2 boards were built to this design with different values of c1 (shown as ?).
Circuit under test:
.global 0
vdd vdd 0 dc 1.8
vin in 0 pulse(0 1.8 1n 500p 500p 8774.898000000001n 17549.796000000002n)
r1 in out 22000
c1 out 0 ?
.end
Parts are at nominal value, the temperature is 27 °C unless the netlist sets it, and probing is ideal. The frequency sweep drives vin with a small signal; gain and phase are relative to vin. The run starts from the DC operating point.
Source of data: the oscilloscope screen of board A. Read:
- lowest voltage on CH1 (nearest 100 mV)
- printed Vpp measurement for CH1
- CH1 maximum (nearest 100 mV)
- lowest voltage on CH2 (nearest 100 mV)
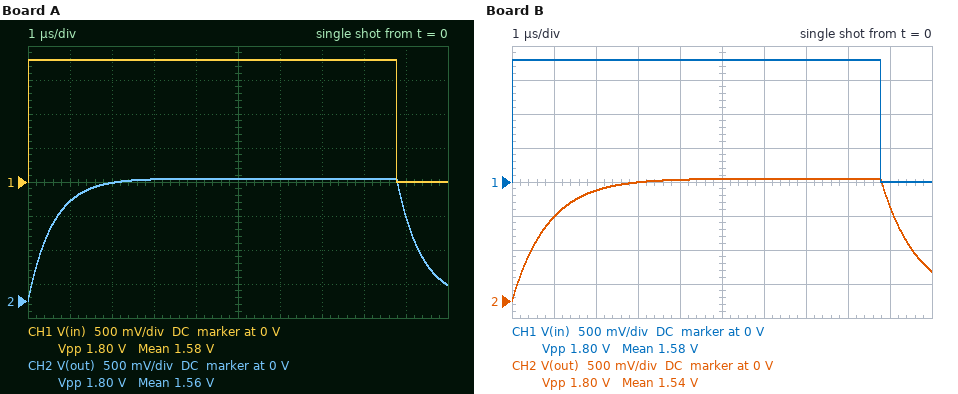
0 V
1.80 V
1.8 V
0 V
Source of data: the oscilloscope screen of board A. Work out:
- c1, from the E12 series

27 pF
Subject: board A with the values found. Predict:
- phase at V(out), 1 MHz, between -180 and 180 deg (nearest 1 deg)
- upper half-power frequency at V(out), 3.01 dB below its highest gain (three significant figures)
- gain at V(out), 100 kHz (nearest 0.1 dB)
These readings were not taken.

-75 deg
268 kHz
-0.6 dB
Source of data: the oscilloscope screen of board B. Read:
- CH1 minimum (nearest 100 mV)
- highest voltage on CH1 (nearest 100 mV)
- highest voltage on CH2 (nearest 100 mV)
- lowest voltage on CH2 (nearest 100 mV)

0 V
1.8 V
1.8 V
0 V
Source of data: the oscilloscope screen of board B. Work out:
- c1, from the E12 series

39 pF
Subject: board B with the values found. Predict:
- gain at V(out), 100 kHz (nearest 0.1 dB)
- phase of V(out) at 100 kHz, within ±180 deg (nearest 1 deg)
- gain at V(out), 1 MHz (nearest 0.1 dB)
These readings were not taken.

-1.1 dB
-28 deg
-14.8 dB
